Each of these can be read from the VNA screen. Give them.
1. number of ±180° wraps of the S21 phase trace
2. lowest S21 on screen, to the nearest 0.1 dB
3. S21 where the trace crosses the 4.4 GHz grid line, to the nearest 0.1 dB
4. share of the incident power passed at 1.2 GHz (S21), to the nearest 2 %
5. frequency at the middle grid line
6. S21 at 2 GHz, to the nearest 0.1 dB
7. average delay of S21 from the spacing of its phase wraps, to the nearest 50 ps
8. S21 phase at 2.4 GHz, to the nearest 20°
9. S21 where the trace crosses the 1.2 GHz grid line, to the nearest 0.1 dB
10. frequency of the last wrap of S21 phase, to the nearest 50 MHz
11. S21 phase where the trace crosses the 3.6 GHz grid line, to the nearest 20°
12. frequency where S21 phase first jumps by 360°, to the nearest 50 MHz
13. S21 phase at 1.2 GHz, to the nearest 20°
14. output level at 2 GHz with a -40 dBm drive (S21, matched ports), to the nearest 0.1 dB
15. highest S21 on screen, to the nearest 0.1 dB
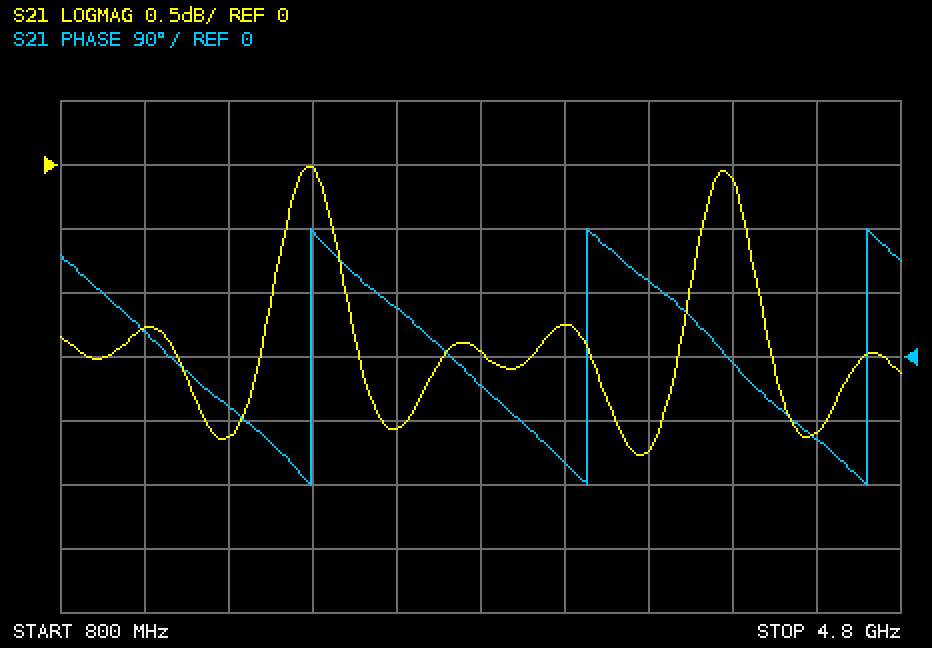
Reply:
3
-2.3 dB
-2.1 dB
74 %
2.8 GHz
0.0 dB
750 ps
60°
-1.3 dB
4.65 GHz
100°
2.00 GHz
40°
-40.0 dBm
0.0 dB
